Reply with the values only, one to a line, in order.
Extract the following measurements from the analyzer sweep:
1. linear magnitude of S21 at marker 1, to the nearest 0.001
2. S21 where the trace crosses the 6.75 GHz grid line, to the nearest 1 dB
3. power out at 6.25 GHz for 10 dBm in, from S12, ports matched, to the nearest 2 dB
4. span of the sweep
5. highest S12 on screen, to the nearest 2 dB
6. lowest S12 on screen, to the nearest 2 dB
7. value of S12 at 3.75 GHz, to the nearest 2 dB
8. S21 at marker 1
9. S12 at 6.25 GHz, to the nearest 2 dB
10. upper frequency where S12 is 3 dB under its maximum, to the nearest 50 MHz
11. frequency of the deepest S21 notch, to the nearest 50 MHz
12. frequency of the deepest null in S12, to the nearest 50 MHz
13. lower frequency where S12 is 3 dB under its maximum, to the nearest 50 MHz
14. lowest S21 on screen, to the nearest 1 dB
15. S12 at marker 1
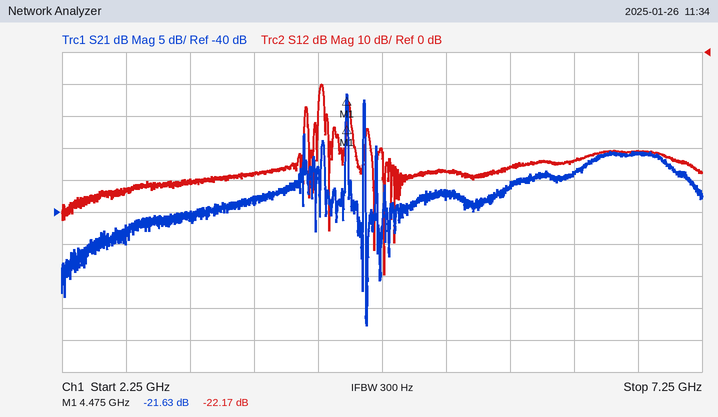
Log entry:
0.083
-31 dB
-24 dBm
5 GHz
-10 dB
-70 dB
-38 dB
-21.63 dB
-34 dB
4.30 GHz
4.65 GHz
4.75 GHz
4.25 GHz
-58 dB
-22.17 dB
